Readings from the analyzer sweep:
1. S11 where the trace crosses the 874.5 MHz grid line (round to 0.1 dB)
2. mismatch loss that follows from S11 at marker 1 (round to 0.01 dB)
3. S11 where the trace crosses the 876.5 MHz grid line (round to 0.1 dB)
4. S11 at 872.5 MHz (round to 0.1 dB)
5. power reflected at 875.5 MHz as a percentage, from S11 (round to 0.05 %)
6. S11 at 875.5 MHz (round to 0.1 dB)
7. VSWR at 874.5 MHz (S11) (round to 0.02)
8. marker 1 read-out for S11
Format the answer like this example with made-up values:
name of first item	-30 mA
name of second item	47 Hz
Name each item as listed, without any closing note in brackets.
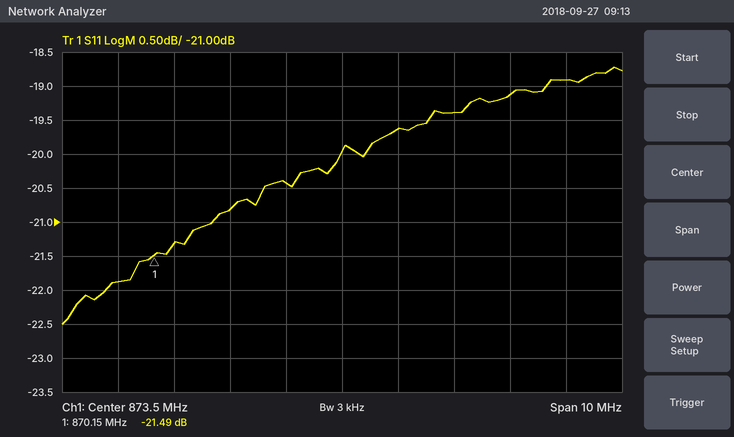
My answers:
S11 where the trace crosses the 874.5 MHz grid line	-19.6 dB
mismatch loss that follows from S11 at marker 1	0.03 dB
S11 where the trace crosses the 876.5 MHz grid line	-19.1 dB
S11 at 872.5 MHz	-20.4 dB
power reflected at 875.5 MHz as a percentage, from S11	1.15 %
S11 at 875.5 MHz	-19.4 dB
VSWR at 874.5 MHz (S11)	1.24
marker 1 read-out for S11	-21.49 dB
